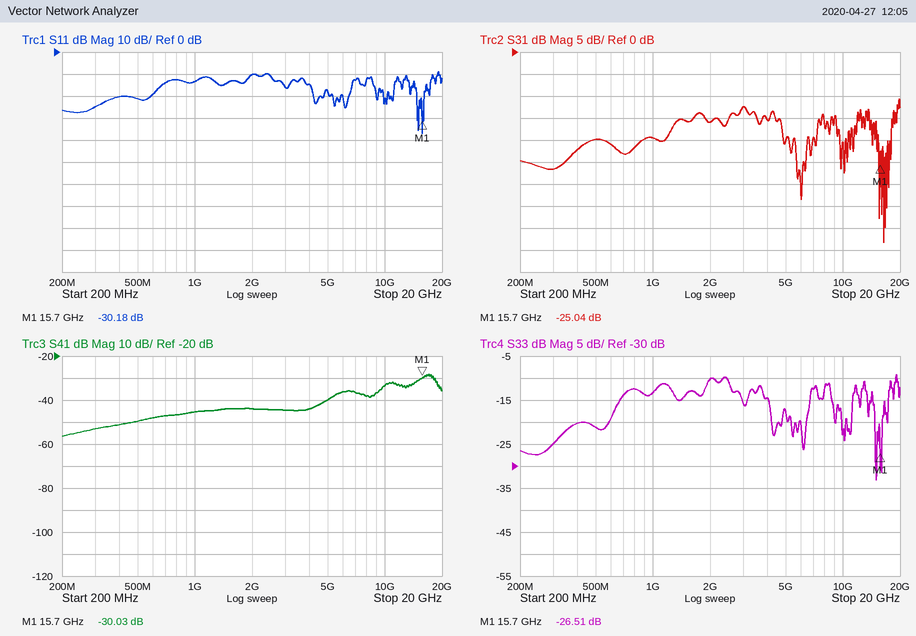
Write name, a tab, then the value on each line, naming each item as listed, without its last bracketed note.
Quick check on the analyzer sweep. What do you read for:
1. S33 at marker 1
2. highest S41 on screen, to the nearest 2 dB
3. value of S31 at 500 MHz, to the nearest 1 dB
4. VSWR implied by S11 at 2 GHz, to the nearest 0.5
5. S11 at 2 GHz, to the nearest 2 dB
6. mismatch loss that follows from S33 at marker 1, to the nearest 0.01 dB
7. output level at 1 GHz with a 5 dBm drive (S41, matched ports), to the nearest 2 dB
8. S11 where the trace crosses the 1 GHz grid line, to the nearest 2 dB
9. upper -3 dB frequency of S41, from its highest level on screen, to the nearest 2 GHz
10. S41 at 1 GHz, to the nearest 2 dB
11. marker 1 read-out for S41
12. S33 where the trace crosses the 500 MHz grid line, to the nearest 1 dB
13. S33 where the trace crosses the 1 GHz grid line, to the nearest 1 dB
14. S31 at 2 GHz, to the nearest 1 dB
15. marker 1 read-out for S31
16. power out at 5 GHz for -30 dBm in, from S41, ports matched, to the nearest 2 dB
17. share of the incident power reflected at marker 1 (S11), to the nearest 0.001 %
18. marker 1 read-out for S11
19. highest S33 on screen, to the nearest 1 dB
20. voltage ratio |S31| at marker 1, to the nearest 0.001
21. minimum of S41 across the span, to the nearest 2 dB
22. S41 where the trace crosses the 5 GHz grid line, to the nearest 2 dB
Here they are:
S33 at marker 1	-26.51 dB
highest S41 on screen, to the nearest 2 dB	-28 dB
value of S31 at 500 MHz, to the nearest 1 dB	-20 dB
VSWR implied by S11 at 2 GHz, to the nearest 0.5	2.0
S11 at 2 GHz, to the nearest 2 dB	-10 dB
mismatch loss that follows from S33 at marker 1, to the nearest 0.01 dB	0.01 dB
output level at 1 GHz with a 5 dBm drive (S41, matched ports), to the nearest 2 dB	-40 dBm
S11 where the trace crosses the 1 GHz grid line, to the nearest 2 dB	-14 dB
upper -3 dB frequency of S41, from its highest level on screen, to the nearest 2 GHz	18 GHz
S41 at 1 GHz, to the nearest 2 dB	-46 dB
marker 1 read-out for S41	-30.03 dB
S33 where the trace crosses the 500 MHz grid line, to the nearest 1 dB	-21 dB
S33 where the trace crosses the 1 GHz grid line, to the nearest 1 dB	-13 dB
S31 at 2 GHz, to the nearest 1 dB	-16 dB
marker 1 read-out for S31	-25.04 dB
power out at 5 GHz for -30 dBm in, from S41, ports matched, to the nearest 2 dB	-70 dBm
share of the incident power reflected at marker 1 (S11), to the nearest 0.001 %	0.096 %
marker 1 read-out for S11	-30.18 dB
highest S33 on screen, to the nearest 1 dB	-9 dB
voltage ratio |S31| at marker 1, to the nearest 0.001	0.056
minimum of S41 across the span, to the nearest 2 dB	-56 dB
S41 where the trace crosses the 5 GHz grid line, to the nearest 2 dB	-40 dB
